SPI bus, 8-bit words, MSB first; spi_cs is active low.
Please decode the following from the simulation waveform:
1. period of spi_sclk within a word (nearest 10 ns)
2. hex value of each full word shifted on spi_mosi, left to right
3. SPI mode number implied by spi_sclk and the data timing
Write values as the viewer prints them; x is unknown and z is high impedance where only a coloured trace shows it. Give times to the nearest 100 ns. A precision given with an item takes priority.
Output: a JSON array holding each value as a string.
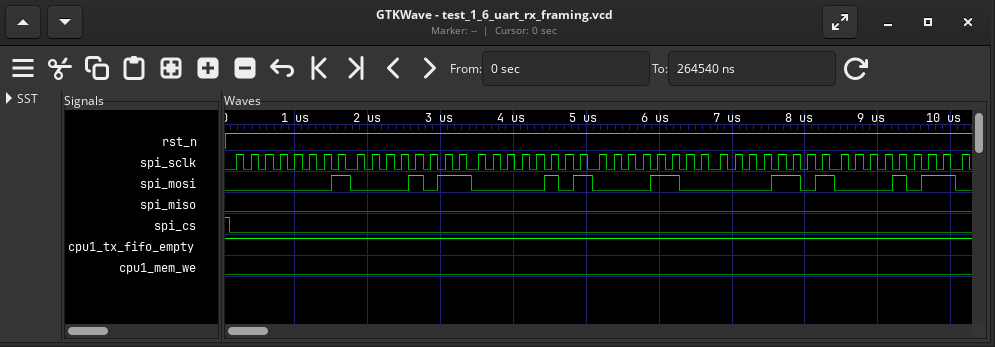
["200 ns", "01, 0B, 05, 0C, 0D, 0B", "0"]
